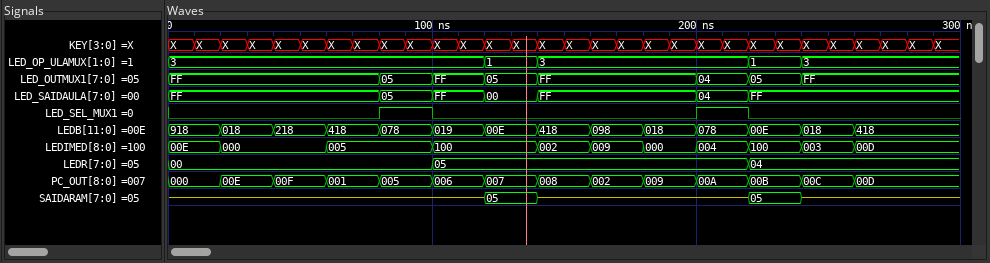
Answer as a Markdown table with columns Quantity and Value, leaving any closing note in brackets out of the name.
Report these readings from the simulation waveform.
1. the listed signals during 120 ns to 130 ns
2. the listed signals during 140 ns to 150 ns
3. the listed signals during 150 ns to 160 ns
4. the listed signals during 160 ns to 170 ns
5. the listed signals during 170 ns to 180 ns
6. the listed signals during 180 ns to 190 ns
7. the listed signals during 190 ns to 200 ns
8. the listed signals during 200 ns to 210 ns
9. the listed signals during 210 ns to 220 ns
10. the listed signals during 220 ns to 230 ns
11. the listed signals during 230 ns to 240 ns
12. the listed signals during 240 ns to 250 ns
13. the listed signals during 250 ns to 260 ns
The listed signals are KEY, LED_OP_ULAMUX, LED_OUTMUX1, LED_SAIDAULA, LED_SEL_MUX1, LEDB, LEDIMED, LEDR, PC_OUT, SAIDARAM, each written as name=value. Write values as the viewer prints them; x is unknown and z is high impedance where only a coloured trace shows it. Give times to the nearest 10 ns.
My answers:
| Quantity | Value |
|---|---|
| the listed signals during 120 ns to 130 ns | KEY=X, LED_OP_ULAMUX=1, LED_OUTMUX1=05, LED_SAIDAULA=00, LED_SEL_MUX1=0, LEDB=00E, LEDIMED=100, LEDR=05, PC_OUT=007, SAIDARAM=05 |
| the listed signals during 140 ns to 150 ns | KEY=X, LED_OP_ULAMUX=3, LED_OUTMUX1=FF, LED_SAIDAULA=FF, LED_SEL_MUX1=0, LEDB=418, LEDIMED=002, LEDR=05, PC_OUT=008, SAIDARAM=z |
| the listed signals during 150 ns to 160 ns | KEY=X, LED_OP_ULAMUX=3, LED_OUTMUX1=FF, LED_SAIDAULA=FF, LED_SEL_MUX1=0, LEDB=418, LEDIMED=002, LEDR=05, PC_OUT=008, SAIDARAM=z |
| the listed signals during 160 ns to 170 ns | KEY=X, LED_OP_ULAMUX=3, LED_OUTMUX1=FF, LED_SAIDAULA=FF, LED_SEL_MUX1=0, LEDB=098, LEDIMED=009, LEDR=05, PC_OUT=002, SAIDARAM=z |
| the listed signals during 170 ns to 180 ns | KEY=X, LED_OP_ULAMUX=3, LED_OUTMUX1=FF, LED_SAIDAULA=FF, LED_SEL_MUX1=0, LEDB=098, LEDIMED=009, LEDR=05, PC_OUT=002, SAIDARAM=z |
| the listed signals during 180 ns to 190 ns | KEY=X, LED_OP_ULAMUX=3, LED_OUTMUX1=FF, LED_SAIDAULA=FF, LED_SEL_MUX1=0, LEDB=018, LEDIMED=000, LEDR=05, PC_OUT=009, SAIDARAM=z |
| the listed signals during 190 ns to 200 ns | KEY=X, LED_OP_ULAMUX=3, LED_OUTMUX1=FF, LED_SAIDAULA=FF, LED_SEL_MUX1=0, LEDB=018, LEDIMED=000, LEDR=05, PC_OUT=009, SAIDARAM=z |
| the listed signals during 200 ns to 210 ns | KEY=X, LED_OP_ULAMUX=3, LED_OUTMUX1=04, LED_SAIDAULA=04, LED_SEL_MUX1=1, LEDB=078, LEDIMED=004, LEDR=05, PC_OUT=00A, SAIDARAM=z |
| the listed signals during 210 ns to 220 ns | KEY=X, LED_OP_ULAMUX=3, LED_OUTMUX1=04, LED_SAIDAULA=04, LED_SEL_MUX1=1, LEDB=078, LEDIMED=004, LEDR=05, PC_OUT=00A, SAIDARAM=z |
| the listed signals during 220 ns to 230 ns | KEY=X, LED_OP_ULAMUX=1, LED_OUTMUX1=05, LED_SAIDAULA=FF, LED_SEL_MUX1=0, LEDB=00E, LEDIMED=100, LEDR=04, PC_OUT=00B, SAIDARAM=05 |
| the listed signals during 230 ns to 240 ns | KEY=X, LED_OP_ULAMUX=1, LED_OUTMUX1=05, LED_SAIDAULA=FF, LED_SEL_MUX1=0, LEDB=00E, LEDIMED=100, LEDR=04, PC_OUT=00B, SAIDARAM=05 |
| the listed signals during 240 ns to 250 ns | KEY=X, LED_OP_ULAMUX=3, LED_OUTMUX1=FF, LED_SAIDAULA=FF, LED_SEL_MUX1=0, LEDB=018, LEDIMED=003, LEDR=04, PC_OUT=00C, SAIDARAM=z |
| the listed signals during 250 ns to 260 ns | KEY=X, LED_OP_ULAMUX=3, LED_OUTMUX1=FF, LED_SAIDAULA=FF, LED_SEL_MUX1=0, LEDB=018, LEDIMED=003, LEDR=04, PC_OUT=00C, SAIDARAM=z |
